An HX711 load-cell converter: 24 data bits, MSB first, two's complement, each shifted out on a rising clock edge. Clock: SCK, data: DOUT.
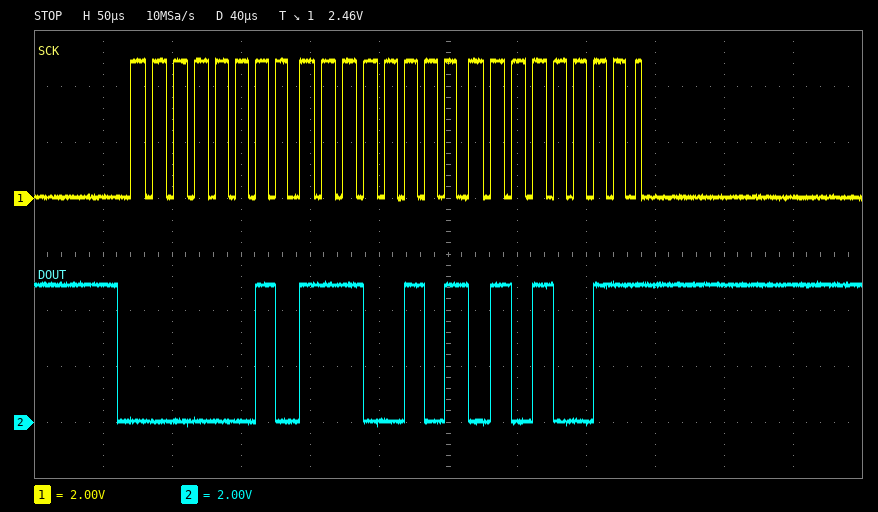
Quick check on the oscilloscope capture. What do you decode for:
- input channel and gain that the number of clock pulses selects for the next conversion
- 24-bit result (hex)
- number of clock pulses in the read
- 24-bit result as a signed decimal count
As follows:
channel A, gain 128
0x02E553
25
189779
